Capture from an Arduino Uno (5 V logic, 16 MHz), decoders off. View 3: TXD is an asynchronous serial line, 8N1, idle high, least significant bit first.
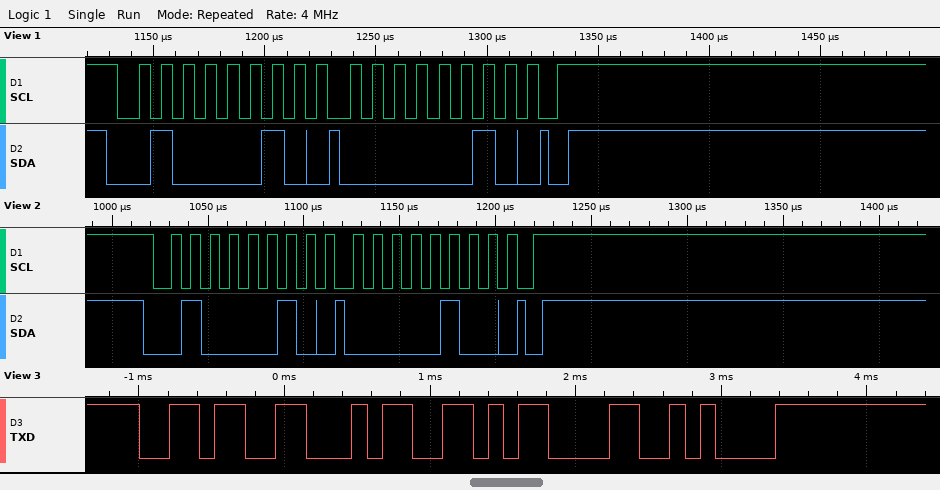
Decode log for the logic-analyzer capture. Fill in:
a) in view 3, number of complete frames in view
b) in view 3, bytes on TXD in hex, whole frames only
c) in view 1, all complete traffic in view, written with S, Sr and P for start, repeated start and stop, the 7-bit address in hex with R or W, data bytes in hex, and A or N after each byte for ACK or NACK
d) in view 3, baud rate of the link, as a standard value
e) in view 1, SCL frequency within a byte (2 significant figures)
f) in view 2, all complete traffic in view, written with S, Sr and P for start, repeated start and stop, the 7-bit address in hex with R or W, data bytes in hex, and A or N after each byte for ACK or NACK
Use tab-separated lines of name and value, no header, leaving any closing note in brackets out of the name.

in view 3, number of complete frames in view	4
in view 3, bytes on TXD in hex, whole frames only	0x36 0x34 0x0D 0x0A
in view 1, all complete traffic in view, written with S, Sr and P for start, repeated start and stop, the 7-bit address in hex with R or W, data bytes in hex, and A or N after each byte for ACK or NACK	S 21W A 02 A P
in view 3, baud rate of the link, as a standard value	9600 baud
in view 1, SCL frequency within a byte	100 kHz
in view 2, all complete traffic in view, written with S, Sr and P for start, repeated start and stop, the 7-bit address in hex with R or W, data bytes in hex, and A or N after each byte for ACK or NACK	S 21W A 04 A P
